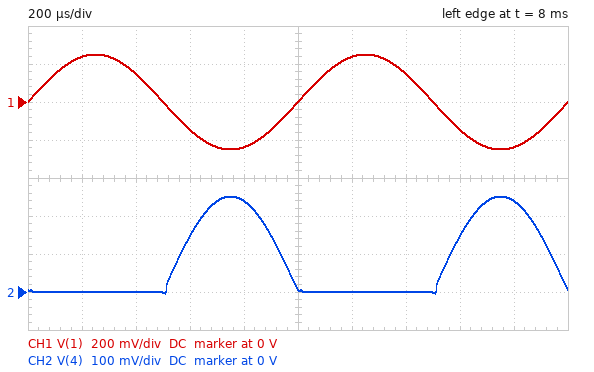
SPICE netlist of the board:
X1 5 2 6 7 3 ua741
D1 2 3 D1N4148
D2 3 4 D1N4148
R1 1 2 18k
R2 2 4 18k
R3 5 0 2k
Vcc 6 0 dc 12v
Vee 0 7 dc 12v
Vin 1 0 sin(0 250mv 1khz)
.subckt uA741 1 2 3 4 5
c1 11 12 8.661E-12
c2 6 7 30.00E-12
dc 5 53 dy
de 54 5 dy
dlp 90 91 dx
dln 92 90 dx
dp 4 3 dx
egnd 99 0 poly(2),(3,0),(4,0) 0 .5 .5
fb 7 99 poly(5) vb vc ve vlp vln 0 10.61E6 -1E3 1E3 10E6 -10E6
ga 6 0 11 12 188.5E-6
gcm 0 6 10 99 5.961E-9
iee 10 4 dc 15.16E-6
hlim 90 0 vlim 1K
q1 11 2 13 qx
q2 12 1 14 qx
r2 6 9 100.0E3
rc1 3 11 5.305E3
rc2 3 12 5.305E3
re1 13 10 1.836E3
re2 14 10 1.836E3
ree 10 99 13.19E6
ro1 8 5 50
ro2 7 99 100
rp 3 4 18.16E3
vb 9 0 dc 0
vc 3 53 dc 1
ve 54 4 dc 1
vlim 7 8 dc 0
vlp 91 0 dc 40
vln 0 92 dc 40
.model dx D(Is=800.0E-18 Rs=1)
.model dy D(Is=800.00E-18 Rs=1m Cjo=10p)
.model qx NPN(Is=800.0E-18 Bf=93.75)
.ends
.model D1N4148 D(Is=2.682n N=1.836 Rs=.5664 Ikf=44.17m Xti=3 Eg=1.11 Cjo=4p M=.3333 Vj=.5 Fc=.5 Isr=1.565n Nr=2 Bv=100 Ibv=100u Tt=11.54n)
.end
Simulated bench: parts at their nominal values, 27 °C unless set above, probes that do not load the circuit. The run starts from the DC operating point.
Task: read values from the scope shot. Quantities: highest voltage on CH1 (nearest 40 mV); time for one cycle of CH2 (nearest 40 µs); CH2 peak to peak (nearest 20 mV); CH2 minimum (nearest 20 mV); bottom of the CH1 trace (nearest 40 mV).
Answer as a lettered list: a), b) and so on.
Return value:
a) 240 mV
b) 1.00 ms
c) 260 mV
d) 0 V
e) -240 mV
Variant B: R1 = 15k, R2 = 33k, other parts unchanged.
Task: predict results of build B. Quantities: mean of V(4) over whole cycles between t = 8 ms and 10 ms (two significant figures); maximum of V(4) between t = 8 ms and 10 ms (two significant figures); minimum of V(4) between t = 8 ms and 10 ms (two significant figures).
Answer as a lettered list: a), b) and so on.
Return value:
a) 180 mV
b) 550 mV
c) -1.5 mV
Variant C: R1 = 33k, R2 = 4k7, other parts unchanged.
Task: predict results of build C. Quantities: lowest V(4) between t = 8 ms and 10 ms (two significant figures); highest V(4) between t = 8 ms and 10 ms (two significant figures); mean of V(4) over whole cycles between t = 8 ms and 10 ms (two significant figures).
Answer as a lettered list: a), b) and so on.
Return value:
a) -5.5 mV
b) 36 mV
c) 11 mV
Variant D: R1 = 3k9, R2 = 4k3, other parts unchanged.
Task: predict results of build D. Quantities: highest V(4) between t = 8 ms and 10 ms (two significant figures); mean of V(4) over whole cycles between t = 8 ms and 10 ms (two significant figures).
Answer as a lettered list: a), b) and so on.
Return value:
a) 280 mV
b) 88 mV
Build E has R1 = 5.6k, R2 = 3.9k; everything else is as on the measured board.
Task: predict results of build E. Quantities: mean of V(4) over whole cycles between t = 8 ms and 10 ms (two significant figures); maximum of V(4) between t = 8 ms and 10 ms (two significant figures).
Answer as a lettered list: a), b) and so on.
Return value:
a) 55 mV
b) 170 mV
